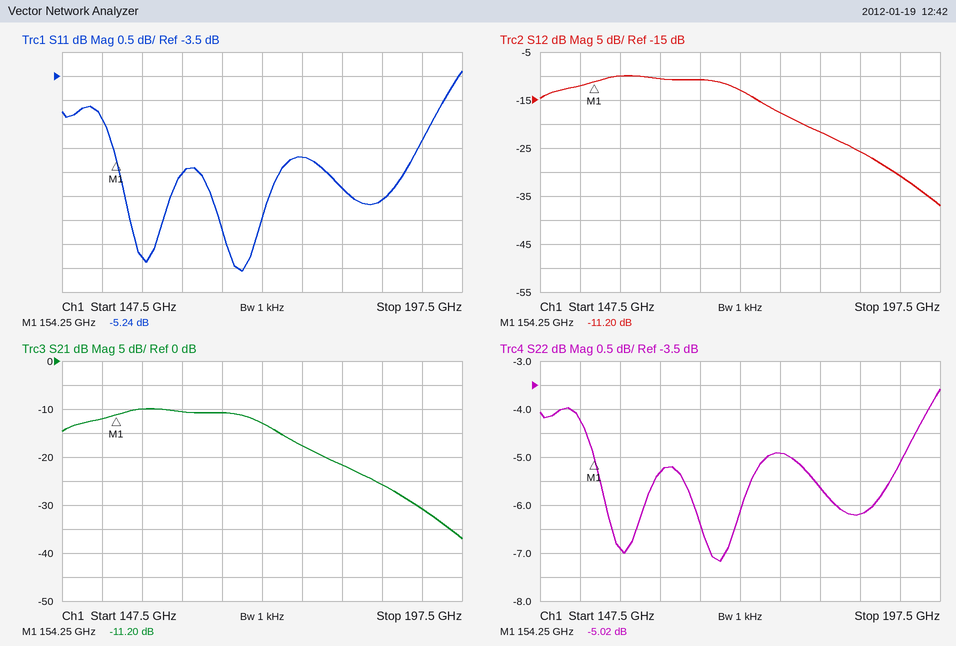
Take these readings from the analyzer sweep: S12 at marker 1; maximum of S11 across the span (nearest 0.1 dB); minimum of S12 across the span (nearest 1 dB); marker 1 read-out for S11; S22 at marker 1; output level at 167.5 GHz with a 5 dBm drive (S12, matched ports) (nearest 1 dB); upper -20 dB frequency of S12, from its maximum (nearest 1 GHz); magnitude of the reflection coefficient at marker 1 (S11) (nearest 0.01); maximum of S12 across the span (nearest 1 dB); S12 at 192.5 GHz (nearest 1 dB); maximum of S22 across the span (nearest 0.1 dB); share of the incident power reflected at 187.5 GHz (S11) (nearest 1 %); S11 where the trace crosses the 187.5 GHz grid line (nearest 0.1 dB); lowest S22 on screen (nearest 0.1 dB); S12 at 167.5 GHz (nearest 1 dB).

-11.20 dB
-3.4 dB
-37 dB
-5.24 dB
-5.02 dB
-6 dBm
192 GHz
0.55
-10 dB
-31 dB
-3.6 dB
25 %
-6.1 dB
-7.2 dB
-11 dB
